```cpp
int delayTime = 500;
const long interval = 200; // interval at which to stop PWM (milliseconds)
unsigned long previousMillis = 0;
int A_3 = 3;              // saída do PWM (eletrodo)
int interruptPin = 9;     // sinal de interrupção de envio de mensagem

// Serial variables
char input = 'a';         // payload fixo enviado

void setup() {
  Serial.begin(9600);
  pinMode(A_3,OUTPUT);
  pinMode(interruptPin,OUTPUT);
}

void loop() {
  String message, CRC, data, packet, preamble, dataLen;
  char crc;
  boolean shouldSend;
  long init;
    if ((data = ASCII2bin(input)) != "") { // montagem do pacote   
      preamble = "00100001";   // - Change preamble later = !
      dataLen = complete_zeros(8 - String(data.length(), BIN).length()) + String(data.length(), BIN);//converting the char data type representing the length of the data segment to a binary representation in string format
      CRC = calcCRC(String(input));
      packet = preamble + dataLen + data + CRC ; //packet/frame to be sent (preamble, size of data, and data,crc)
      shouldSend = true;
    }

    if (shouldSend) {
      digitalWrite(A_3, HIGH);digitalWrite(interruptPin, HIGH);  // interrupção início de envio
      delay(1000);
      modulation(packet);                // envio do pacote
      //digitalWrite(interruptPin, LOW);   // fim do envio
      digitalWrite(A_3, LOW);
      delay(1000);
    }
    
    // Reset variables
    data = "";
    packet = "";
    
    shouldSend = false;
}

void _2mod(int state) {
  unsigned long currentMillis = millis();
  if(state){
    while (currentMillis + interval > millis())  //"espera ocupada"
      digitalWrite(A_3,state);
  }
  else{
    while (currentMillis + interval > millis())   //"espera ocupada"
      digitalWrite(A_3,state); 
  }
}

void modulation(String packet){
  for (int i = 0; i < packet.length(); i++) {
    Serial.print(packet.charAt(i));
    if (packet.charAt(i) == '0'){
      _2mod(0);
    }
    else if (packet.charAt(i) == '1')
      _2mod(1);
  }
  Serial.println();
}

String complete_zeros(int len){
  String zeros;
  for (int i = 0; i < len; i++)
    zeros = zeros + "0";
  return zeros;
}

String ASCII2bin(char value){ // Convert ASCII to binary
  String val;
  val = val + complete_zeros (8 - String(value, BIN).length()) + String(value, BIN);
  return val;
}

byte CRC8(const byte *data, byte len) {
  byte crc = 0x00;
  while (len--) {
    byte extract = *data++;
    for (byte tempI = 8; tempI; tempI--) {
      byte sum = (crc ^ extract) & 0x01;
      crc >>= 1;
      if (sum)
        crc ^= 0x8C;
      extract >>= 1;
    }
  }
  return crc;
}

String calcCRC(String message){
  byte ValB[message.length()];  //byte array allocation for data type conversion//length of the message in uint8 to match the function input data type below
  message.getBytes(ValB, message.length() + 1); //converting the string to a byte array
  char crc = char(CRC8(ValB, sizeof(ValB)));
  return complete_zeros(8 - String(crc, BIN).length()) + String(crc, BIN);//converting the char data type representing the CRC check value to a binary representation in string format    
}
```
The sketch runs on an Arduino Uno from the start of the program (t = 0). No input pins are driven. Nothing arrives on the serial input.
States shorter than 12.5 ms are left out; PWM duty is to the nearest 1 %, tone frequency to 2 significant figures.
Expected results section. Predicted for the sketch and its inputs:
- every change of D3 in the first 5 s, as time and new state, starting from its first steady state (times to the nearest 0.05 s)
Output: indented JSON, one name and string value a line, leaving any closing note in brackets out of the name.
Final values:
{
  "every change of D3 in the first 5 s, as time and new state, starting from its first steady state": "0 s high; 1 s low; 1.4 s high; 1.6 s low; 2.4 s high; 2.6 s low; 3.4 s high; 3.6 s low; 4.4 s high; 4.8 s low"
}
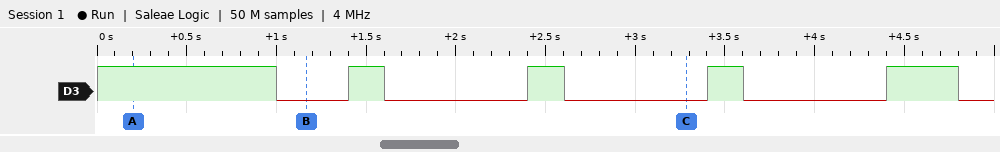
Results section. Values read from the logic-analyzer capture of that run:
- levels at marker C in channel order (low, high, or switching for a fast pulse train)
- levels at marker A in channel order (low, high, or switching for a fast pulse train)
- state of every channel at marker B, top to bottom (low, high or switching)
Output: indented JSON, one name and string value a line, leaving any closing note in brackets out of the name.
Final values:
{
  "levels at marker C in channel order": "D3 low",
  "levels at marker A in channel order": "D3 high",
  "state of every channel at marker B, top to bottom": "D3 low"
}
